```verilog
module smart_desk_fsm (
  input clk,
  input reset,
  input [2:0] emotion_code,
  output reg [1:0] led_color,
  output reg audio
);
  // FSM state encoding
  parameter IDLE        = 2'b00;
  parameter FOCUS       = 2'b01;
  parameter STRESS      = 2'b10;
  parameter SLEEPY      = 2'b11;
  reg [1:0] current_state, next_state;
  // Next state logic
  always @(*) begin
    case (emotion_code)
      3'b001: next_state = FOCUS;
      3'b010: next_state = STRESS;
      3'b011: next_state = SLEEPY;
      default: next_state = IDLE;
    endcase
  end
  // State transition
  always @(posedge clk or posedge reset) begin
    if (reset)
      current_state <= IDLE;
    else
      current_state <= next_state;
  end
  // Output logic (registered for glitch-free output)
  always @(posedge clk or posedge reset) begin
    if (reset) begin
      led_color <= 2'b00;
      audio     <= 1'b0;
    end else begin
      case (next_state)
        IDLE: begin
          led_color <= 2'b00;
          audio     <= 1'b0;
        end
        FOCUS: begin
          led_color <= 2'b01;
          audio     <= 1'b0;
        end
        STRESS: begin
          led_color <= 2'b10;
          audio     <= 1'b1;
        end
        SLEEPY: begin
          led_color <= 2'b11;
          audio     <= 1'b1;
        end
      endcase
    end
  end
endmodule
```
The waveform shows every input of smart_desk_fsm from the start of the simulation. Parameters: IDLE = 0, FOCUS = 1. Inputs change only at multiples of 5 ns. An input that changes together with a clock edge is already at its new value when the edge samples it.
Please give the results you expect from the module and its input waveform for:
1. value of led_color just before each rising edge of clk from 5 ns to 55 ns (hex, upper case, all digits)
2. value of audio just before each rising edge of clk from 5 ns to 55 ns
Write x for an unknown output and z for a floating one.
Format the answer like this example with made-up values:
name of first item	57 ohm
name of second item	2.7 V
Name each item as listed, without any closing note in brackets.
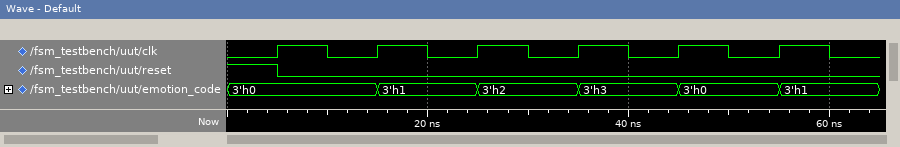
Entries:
value of led_color just before each rising edge of clk from 5 ns to 55 ns	0, 0, 1, 2, 3, 0
value of audio just before each rising edge of clk from 5 ns to 55 ns	0 0 0 1 1 0
